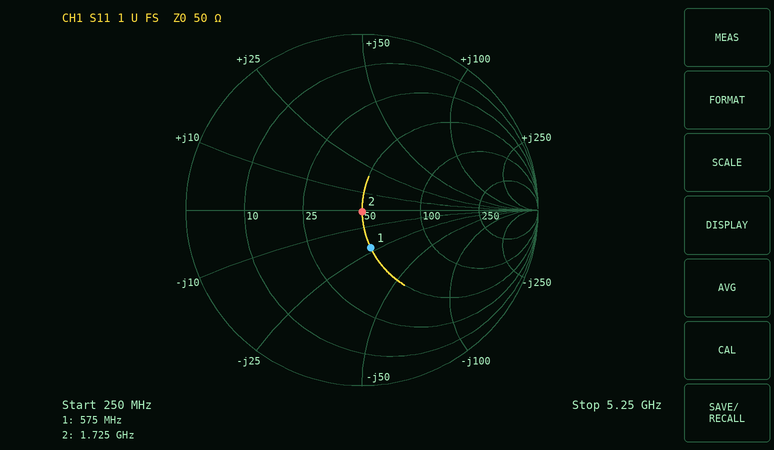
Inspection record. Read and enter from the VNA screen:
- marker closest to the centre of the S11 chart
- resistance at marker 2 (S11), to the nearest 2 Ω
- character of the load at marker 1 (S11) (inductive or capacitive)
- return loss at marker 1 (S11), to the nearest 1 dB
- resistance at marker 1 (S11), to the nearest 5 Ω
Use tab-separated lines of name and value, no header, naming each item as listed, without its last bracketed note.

marker closest to the centre of the S11 chart	marker 2
resistance at marker 2 (S11), to the nearest 2 Ω	50 Ω
character of the load at marker 1 (S11)	capacitive
return loss at marker 1 (S11), to the nearest 1 dB	13 dB
resistance at marker 1 (S11), to the nearest 5 Ω	50 Ω
